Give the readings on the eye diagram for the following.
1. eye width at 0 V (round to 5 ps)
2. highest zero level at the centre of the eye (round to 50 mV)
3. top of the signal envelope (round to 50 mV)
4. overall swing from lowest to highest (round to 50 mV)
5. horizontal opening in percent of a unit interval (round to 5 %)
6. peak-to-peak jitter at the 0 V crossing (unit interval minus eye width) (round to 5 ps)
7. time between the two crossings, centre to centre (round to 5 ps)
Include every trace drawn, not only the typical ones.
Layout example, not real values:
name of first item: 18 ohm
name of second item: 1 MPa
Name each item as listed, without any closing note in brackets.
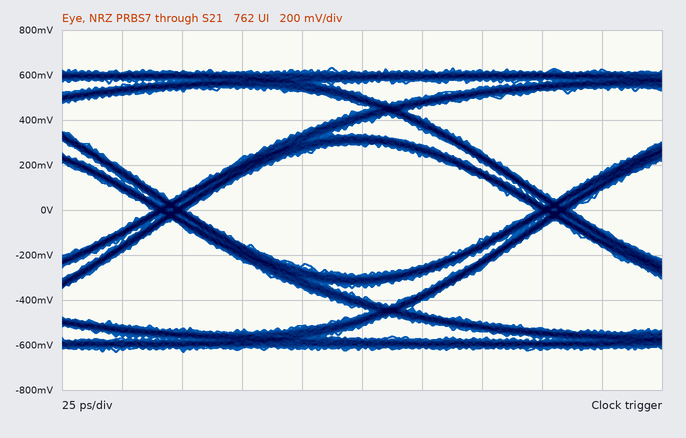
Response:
eye width at 0 V: 145 ps
highest zero level at the centre of the eye: -300 mV
top of the signal envelope: 650 mV
overall swing from lowest to highest: 1.25 V
horizontal opening in percent of a unit interval: 90 %
peak-to-peak jitter at the 0 V crossing (unit interval minus eye width): 15 ps
time between the two crossings, centre to centre: 160 ps
